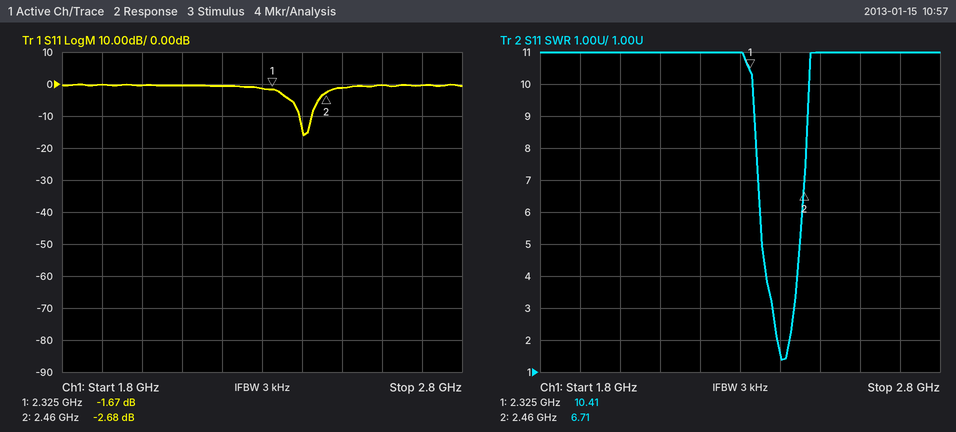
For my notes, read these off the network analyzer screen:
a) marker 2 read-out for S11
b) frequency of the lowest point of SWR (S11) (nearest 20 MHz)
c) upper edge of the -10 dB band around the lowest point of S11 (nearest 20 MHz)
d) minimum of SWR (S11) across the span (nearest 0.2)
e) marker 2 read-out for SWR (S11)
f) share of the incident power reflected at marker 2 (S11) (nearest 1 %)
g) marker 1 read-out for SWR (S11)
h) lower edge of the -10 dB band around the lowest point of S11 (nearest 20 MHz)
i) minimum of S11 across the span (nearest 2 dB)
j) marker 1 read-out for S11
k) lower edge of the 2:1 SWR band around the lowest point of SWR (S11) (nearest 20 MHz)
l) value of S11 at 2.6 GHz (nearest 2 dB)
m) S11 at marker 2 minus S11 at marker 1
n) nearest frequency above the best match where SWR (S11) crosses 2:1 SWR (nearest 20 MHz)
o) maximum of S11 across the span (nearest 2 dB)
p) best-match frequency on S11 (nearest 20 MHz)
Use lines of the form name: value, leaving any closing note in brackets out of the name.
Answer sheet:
marker 2 read-out for S11: -2.68 dB
frequency of the lowest point of SWR (S11): 2.40 GHz
upper edge of the -10 dB band around the lowest point of S11: 2.42 GHz
minimum of SWR (S11) across the span: 1.4
marker 2 read-out for SWR: 6.71
share of the incident power reflected at marker 2 (S11): 54 %
marker 1 read-out for SWR: 10.41
lower edge of the -10 dB band around the lowest point of S11: 2.40 GHz
minimum of S11 across the span: -16 dB
marker 1 read-out for S11: -1.67 dB
lower edge of the 2:1 SWR band around the lowest point of SWR (S11): 2.40 GHz
value of S11 at 2.6 GHz: 0 dB
S11 at marker 2 minus S11 at marker 1: -1.01 dB
nearest frequency above the best match where SWR (S11) crosses 2:1 SWR: 2.42 GHz
maximum of S11 across the span: 0 dB
best-match frequency on S11: 2.40 GHz
